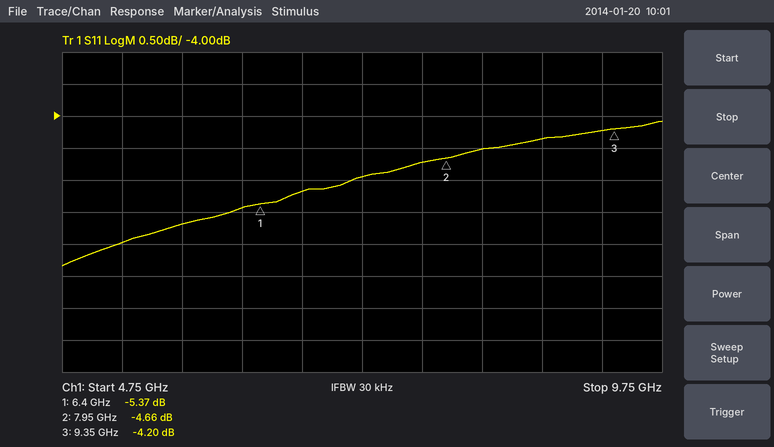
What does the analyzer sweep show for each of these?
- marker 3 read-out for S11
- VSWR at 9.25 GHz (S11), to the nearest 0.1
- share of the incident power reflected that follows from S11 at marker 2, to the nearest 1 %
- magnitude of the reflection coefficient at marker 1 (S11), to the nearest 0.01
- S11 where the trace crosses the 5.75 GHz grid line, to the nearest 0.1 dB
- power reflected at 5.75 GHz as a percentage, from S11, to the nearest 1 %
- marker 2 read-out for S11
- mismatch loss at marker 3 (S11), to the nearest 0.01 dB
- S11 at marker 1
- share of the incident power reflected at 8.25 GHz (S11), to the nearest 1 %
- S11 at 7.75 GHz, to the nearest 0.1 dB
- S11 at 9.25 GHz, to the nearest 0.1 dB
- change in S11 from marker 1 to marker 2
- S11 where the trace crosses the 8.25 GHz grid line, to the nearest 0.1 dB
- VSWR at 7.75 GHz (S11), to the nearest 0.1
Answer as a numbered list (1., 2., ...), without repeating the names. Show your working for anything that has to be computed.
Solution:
1. -4.20 dB
2. |Γ| = 10^(-4.2/20) = 0.6166; VSWR = (1 + 0.6166)/(1 − 0.6166) ≈ 4.2
3. 10^(-4.66/10) ≈ 34 %
4. 10^(-5.37/20) ≈ 0.54
5. -5.7 dB
6. 10^(-5.7/10) ≈ 27 %
7. -4.66 dB
8. −10 log10(1 − 10^(-4.2/10)) ≈ 2.08 dB
9. -5.37 dB
10. 10^(-4.5/10) ≈ 35 %
11. -4.7 dB
12. -4.2 dB
13. -4.66 − (-5.37) = 0.71 dB
14. -4.5 dB
15. |Γ| = 10^(-4.7/20) = 0.5821; VSWR = (1 + 0.5821)/(1 − 0.5821) ≈ 3.8
